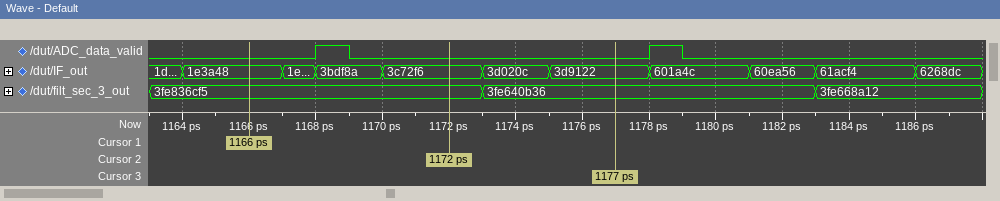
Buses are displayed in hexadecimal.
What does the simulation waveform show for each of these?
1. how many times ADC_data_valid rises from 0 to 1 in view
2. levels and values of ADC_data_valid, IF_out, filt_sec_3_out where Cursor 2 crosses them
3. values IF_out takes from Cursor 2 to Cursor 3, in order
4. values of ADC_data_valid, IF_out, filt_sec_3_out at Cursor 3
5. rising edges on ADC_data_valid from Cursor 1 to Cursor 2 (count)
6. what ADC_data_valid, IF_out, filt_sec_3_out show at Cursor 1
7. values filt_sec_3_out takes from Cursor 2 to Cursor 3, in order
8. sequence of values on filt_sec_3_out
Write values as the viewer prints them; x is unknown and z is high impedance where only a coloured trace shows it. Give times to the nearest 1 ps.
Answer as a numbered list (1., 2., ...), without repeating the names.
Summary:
1. 2
2. ADC_data_valid=0, IF_out=3c72f6, filt_sec_3_out=3fe836cf5
3. 3c72f6, 3d020c, 3d9122
4. ADC_data_valid=0, IF_out=3d9122, filt_sec_3_out=3fe640b36
5. 1
6. ADC_data_valid=0, IF_out=1e3a48, filt_sec_3_out=3fe836cf5
7. 3fe836cf5, 3fe640b36
8. 3fe836cf5, 3fe640b36, 3fe668a12
